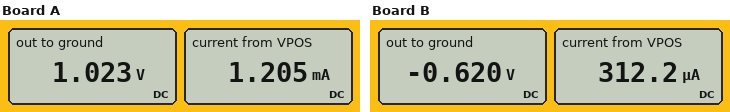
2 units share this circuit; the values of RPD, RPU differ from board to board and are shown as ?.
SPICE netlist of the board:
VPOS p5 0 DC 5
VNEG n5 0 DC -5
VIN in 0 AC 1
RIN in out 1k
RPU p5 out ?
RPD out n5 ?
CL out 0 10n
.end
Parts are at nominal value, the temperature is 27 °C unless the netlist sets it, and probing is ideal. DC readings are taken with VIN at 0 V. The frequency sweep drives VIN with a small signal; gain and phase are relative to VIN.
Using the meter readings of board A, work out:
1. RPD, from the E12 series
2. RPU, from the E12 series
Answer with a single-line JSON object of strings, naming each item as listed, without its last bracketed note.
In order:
{"RPD, from the E12 series": "33 kΩ", "RPU, from the E12 series": "3.3 kΩ"}
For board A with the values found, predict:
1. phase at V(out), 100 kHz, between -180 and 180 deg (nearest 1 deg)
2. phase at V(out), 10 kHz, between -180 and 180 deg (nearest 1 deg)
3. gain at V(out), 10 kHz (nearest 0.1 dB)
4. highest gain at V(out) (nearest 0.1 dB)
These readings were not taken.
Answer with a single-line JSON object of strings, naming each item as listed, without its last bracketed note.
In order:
{"phase at V(out), 100 kHz, between -180 and 180 deg": "-78 deg", "phase at V(out), 10 kHz, between -180 and 180 deg": "-25 deg", "gain at V(out), 10 kHz": "-3.4 dB", "highest gain at V(out)": "-2.5 dB"}
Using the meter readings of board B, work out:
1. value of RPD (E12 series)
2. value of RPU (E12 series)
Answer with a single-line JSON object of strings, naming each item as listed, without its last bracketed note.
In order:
{"value of RPD": "4.7 kΩ", "value of RPU": "18 kΩ"}
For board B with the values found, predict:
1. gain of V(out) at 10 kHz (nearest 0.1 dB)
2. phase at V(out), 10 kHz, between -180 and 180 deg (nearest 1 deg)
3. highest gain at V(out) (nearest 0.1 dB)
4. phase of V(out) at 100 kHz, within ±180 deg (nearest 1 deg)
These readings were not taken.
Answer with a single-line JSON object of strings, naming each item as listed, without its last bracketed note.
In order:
{"gain of V(out) at 10 kHz": "-3.0 dB", "phase at V(out), 10 kHz, between -180 and 180 deg": "-26 deg", "highest gain at V(out)": "-2.1 dB", "phase of V(out) at 100 kHz, within ±180 deg": "-79 deg"}
